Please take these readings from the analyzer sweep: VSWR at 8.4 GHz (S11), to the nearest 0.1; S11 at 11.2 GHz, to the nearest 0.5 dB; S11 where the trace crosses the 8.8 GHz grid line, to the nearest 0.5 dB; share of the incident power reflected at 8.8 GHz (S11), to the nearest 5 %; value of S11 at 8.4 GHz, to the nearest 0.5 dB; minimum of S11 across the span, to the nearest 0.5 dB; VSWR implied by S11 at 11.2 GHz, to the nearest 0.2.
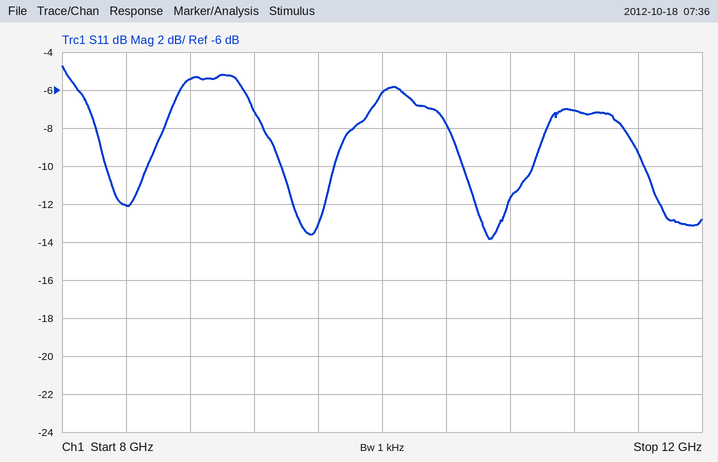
1.7
-7.0 dB
-5.5 dB
30 %
-12.0 dB
-14.0 dB
2.6
